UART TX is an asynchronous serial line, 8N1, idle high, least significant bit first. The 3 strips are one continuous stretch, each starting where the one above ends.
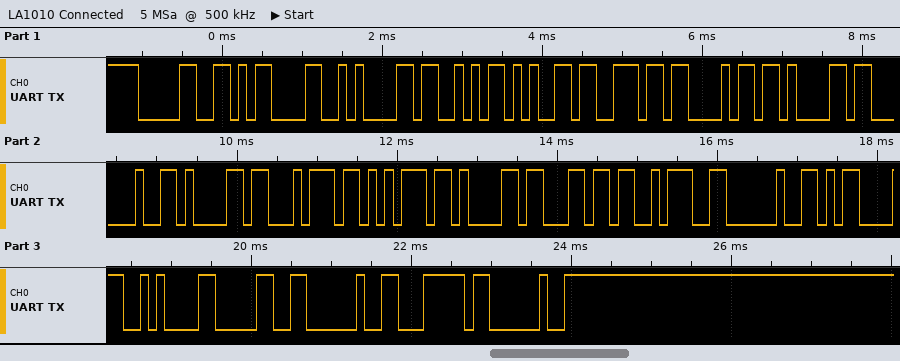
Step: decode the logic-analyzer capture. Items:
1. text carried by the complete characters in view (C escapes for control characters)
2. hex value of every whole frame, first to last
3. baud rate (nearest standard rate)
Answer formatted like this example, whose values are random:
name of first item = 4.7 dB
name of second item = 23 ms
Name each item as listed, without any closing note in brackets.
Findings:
text carried by the complete characters in view = "0\r\nSenha atual: \r\n0 | "
hex value of every whole frame, first to last = 30 0D 0A 53 65 6E 68 61 20 61 74 75 61 6C 3A 20 0D 0A 30 20 7C 20
baud rate = 9600 baud
